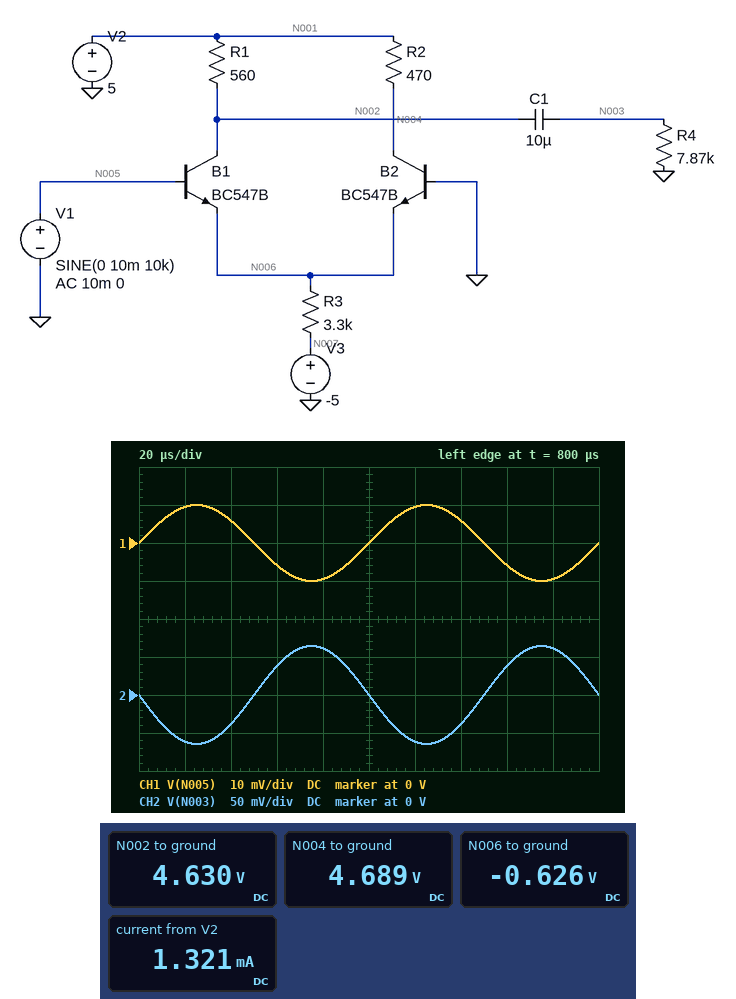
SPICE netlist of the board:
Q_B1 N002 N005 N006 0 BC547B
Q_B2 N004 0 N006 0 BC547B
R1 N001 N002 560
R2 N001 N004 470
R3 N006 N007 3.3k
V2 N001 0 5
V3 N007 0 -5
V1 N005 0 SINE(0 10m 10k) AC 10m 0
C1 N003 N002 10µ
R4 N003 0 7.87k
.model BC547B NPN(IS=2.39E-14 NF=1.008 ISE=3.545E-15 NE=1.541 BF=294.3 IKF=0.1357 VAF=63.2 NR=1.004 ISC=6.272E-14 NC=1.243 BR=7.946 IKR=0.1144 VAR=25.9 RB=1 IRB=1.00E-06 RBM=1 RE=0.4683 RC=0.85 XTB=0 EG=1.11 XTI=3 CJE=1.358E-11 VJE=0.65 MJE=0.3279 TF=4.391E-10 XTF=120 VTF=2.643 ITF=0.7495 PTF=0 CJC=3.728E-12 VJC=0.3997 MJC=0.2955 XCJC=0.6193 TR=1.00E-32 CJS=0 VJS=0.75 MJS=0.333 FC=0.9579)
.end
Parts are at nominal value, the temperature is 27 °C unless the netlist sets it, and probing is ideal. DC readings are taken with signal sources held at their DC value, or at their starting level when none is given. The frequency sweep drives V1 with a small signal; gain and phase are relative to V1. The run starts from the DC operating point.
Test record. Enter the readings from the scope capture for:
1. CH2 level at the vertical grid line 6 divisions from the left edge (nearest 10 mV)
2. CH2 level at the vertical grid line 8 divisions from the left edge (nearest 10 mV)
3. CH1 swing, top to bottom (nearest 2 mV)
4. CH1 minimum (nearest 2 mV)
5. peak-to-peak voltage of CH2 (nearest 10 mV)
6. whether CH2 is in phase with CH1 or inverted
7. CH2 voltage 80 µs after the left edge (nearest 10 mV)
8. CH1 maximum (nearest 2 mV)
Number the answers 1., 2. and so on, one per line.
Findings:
1. -60 mV
2. 40 mV
3. 20 mV
4. -10 mV
5. 130 mV
6. inverted
7. 60 mV
8. 10 mV
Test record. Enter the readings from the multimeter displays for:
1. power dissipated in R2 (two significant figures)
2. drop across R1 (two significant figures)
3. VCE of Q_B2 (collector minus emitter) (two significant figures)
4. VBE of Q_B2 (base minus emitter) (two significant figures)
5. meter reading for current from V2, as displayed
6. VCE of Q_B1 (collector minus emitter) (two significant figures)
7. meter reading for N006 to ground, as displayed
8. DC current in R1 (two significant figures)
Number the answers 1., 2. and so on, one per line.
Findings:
1. 210 µW
2. 370 mV
3. 5.3 V
4. 630 mV
5. 1.321 mA
6. 5.3 V
7. -0.626 V
8. 660 µA
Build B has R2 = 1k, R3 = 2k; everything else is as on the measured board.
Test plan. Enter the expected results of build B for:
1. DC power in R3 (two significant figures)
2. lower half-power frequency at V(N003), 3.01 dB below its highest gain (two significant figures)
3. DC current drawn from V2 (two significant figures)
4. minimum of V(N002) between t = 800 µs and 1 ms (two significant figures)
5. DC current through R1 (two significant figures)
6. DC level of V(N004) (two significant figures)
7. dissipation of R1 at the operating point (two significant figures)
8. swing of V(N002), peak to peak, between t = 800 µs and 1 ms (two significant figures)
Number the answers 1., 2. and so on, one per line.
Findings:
1. 9.5 mW
2. 1.9 Hz
3. 2.2 mA
4. 4.3 V
5. 1.1 mA
6. 3.9 V
7. 670 µW
8. 210 mV
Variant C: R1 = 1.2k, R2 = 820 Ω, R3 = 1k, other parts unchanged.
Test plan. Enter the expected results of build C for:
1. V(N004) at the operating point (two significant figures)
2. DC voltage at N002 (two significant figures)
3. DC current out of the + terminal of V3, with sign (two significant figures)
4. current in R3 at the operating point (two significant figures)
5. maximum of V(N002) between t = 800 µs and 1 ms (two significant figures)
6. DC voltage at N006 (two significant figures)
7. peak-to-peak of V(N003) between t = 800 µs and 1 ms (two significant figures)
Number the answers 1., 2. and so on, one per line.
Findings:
1. 3.2 V
2. 2.4 V
3. -4.3 mA
4. 4.3 mA
5. 2.8 V
6. -660 mV
7. 790 mV
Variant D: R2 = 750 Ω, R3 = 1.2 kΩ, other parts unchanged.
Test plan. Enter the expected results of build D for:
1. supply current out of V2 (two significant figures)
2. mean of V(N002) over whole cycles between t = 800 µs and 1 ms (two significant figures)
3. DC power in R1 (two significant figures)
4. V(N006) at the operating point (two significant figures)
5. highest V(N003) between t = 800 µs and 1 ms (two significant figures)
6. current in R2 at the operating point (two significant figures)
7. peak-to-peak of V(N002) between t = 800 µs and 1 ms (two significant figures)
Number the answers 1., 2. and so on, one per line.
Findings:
1. 3.6 mA
2. 4.0 V
3. 1.8 mW
4. -650 mV
5. 170 mV
6. 1.8 mA
7. 340 mV
